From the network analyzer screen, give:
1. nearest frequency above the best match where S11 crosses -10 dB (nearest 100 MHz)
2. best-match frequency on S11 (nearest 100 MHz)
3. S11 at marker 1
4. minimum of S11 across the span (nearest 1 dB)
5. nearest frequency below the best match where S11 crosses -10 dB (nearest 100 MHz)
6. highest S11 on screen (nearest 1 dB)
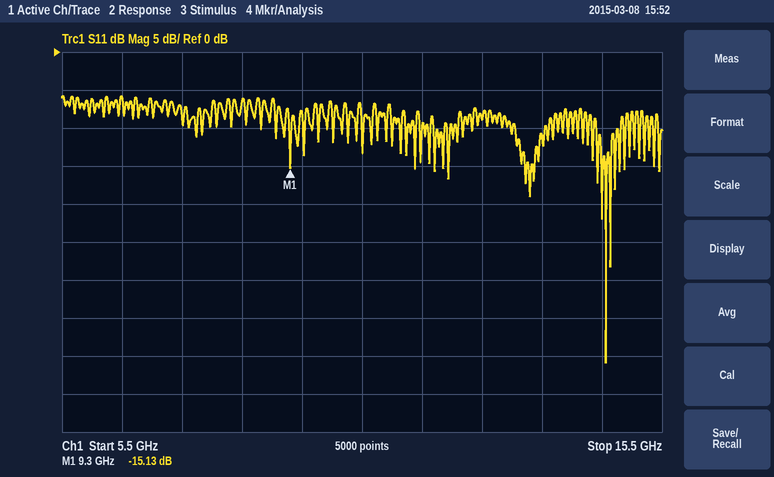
14.8 GHz
14.6 GHz
-15.13 dB
-41 dB
14.4 GHz
-6 dB
